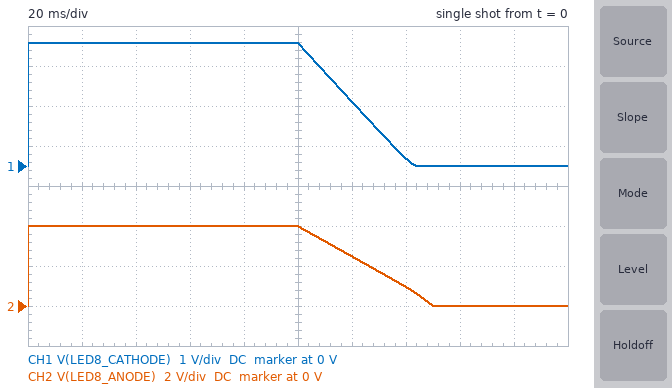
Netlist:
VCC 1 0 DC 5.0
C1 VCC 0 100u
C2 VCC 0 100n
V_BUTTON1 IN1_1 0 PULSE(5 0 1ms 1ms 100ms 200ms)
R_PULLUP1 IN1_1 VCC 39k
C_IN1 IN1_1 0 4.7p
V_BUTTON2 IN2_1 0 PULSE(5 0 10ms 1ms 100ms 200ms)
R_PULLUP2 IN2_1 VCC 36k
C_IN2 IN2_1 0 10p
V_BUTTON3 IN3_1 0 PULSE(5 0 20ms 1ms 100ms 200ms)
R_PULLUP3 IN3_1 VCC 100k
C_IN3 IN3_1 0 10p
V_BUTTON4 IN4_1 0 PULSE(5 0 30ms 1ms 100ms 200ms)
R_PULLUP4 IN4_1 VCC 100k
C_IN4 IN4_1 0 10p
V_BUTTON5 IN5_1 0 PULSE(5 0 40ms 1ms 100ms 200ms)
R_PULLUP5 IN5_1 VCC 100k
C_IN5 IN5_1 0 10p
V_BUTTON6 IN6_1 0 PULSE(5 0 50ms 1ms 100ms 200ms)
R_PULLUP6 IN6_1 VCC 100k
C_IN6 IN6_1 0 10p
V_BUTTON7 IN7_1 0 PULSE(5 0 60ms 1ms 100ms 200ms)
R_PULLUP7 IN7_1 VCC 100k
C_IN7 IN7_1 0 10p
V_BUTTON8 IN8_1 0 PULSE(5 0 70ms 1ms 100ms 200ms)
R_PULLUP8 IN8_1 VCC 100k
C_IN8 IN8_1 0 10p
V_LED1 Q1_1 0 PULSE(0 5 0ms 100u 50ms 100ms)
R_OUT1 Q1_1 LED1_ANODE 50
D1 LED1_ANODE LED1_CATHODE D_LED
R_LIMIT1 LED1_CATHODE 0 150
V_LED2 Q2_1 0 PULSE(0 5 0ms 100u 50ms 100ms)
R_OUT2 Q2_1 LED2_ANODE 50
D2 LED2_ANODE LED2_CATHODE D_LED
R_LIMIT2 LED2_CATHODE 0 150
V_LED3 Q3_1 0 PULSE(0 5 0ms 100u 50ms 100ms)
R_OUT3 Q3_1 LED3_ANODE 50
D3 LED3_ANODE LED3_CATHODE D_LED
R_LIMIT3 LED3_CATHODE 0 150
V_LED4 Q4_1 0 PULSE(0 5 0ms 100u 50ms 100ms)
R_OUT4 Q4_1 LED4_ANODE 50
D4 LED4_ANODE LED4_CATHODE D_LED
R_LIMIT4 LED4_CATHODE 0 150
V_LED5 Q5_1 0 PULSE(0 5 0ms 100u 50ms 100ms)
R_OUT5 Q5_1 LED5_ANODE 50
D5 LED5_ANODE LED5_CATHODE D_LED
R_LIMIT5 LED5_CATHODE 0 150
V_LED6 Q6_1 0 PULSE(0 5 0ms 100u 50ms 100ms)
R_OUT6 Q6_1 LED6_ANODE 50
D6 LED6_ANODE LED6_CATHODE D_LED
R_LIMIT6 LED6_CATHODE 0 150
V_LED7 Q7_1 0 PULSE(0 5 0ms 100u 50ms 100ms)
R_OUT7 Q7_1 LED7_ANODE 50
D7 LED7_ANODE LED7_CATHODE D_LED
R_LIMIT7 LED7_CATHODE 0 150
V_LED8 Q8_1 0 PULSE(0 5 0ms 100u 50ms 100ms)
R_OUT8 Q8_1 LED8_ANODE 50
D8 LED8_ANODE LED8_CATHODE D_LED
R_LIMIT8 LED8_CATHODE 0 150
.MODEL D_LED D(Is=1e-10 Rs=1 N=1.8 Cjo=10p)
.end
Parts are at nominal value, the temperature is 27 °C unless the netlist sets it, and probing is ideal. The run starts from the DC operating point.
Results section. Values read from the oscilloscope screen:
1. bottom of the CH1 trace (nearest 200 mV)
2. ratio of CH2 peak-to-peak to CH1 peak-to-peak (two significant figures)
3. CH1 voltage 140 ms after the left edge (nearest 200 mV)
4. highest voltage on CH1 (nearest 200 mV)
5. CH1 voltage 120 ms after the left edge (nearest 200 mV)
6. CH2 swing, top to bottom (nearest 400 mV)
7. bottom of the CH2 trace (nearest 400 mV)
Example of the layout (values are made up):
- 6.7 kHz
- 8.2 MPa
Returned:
- 0 V
- 1.3
- 200 mV
- 3.0 V
- 1.6 V
- 4.0 V
- 0 V
